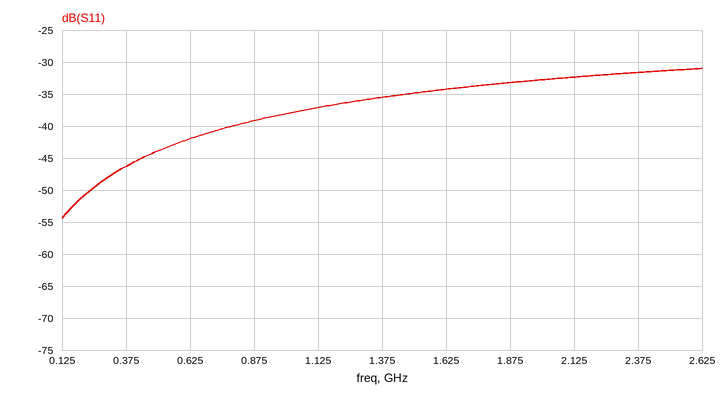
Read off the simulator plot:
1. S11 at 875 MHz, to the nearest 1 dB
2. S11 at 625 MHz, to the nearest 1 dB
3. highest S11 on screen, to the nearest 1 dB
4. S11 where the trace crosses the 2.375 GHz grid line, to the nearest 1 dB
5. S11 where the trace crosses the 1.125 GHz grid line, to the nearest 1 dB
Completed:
-39 dB
-42 dB
-31 dB
-32 dB
-37 dB
